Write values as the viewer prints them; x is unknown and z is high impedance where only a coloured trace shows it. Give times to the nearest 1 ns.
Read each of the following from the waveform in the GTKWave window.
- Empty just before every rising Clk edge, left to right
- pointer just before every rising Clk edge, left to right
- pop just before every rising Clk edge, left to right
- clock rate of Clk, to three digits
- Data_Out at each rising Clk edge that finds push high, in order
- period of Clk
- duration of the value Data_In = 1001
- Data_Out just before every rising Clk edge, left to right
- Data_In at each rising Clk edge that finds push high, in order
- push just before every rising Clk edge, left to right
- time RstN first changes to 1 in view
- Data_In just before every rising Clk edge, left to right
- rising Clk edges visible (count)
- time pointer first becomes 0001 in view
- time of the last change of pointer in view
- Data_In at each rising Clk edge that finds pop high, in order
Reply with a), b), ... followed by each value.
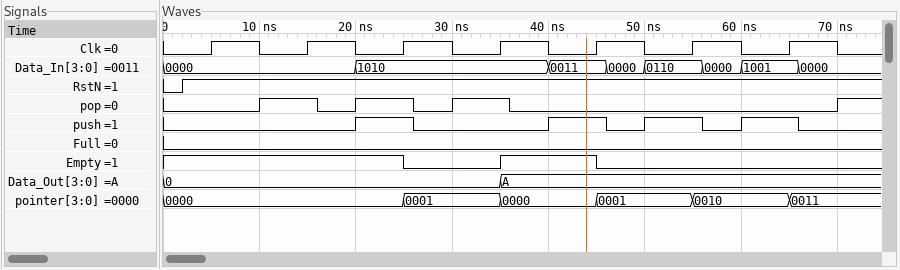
a) 1 1 1 0 1 0 0
b) 0000, 0000, 0000, 0001, 0000, 0001, 0010
c) 0 1 1 1 0 0 0
d) 100 MHz
e) 0, A, A, A
f) 10 ns
g) 6 ns
h) 0, 0, 0, 0, A, A, A
i) 1010, 0011, 0110, 1001
j) 0 0 1 0 1 1 1
k) 2 ns
l) 0000, 0000, 1010, 1010, 0011, 0110, 1001
m) 7
n) 25 ns
o) 65 ns
p) 0000, 1010, 1010
